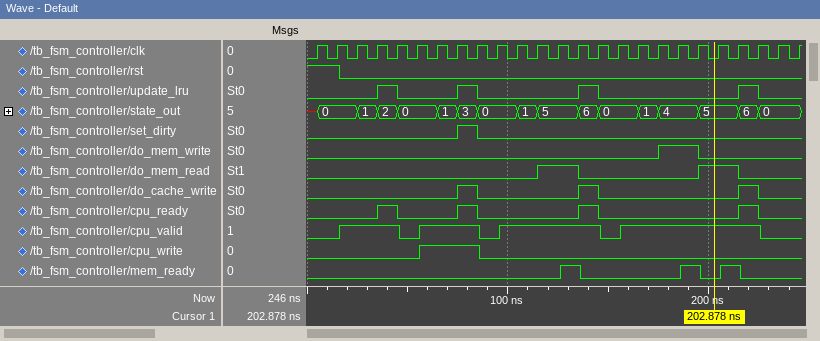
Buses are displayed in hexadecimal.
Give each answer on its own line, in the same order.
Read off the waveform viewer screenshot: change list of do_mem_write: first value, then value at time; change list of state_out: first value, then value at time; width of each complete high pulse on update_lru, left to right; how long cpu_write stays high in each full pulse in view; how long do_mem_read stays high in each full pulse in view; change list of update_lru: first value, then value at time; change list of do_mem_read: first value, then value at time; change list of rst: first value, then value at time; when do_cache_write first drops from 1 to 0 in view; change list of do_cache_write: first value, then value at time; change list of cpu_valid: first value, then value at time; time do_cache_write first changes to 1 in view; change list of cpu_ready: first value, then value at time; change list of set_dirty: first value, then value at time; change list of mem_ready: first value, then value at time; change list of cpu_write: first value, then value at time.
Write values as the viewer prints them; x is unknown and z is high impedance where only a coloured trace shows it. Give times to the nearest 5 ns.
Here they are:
0, 1 at 175 ns, 0 at 195 ns
x, 0 at 5 ns, 1 at 25 ns, 2 at 35 ns, 0 at 45 ns, 1 at 65 ns, 3 at 75 ns, 0 at 85 ns, 1 at 105 ns, 5 at 115 ns, 6 at 135 ns, 0 at 145 ns, 1 at 165 ns, 4 at 175 ns, 5 at 195 ns, 6 at 215 ns, 0 at 225 ns
10 ns, 10 ns, 10 ns, 10 ns
30 ns
20 ns, 20 ns
0, 1 at 35 ns, 0 at 45 ns, 1 at 75 ns, 0 at 85 ns, 1 at 135 ns, 0 at 145 ns, 1 at 215 ns, 0 at 225 ns
0, 1 at 115 ns, 0 at 135 ns, 1 at 195 ns, 0 at 215 ns
1, 0 at 15 ns
85 ns
0, 1 at 75 ns, 0 at 85 ns, 1 at 135 ns, 0 at 145 ns, 1 at 215 ns, 0 at 225 ns
0, 1 at 15 ns, 0 at 45 ns, 1 at 55 ns, 0 at 85 ns, 1 at 95 ns, 0 at 145 ns, 1 at 155 ns, 0 at 225 ns
75 ns
0, 1 at 35 ns, 0 at 45 ns, 1 at 75 ns, 0 at 85 ns, 1 at 135 ns, 0 at 145 ns, 1 at 215 ns, 0 at 225 ns
0, 1 at 75 ns, 0 at 85 ns
0, 1 at 125 ns, 0 at 135 ns, 1 at 185 ns, 0 at 195 ns, 1 at 205 ns, 0 at 215 ns
0, 1 at 55 ns, 0 at 85 ns
